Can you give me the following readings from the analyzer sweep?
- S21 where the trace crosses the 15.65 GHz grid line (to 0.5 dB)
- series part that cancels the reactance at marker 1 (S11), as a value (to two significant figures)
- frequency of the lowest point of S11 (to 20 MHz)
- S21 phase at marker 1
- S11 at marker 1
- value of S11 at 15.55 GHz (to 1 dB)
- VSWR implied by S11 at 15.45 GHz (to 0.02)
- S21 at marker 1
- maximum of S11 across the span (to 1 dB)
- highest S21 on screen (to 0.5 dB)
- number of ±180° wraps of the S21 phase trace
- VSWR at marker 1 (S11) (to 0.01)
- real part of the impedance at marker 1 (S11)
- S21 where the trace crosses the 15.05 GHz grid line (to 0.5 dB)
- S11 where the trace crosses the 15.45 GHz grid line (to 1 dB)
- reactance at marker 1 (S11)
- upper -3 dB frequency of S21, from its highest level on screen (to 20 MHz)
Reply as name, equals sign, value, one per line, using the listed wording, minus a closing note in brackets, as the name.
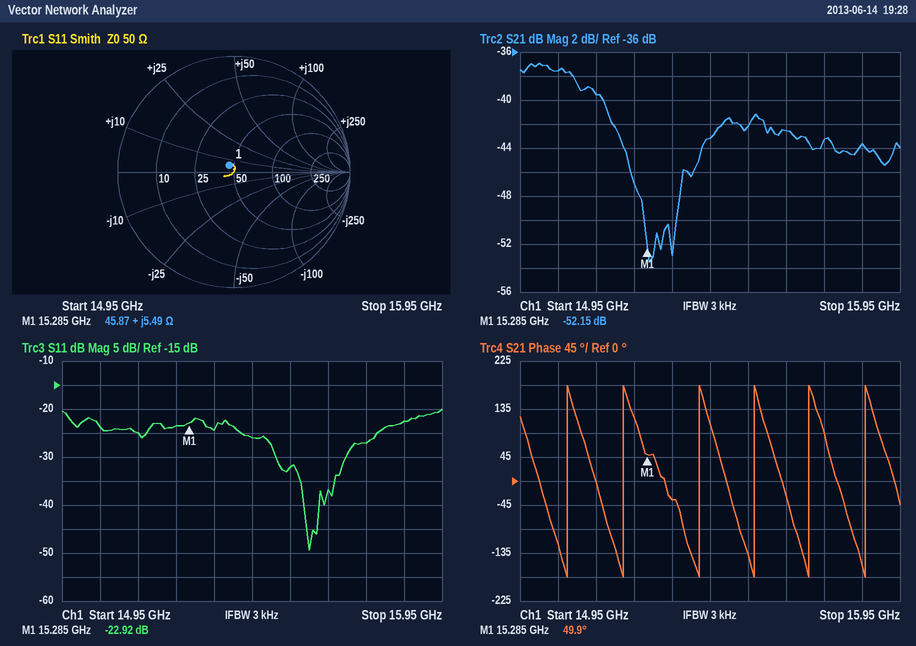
S21 where the trace crosses the 15.65 GHz grid line = -42.5 dB
series part that cancels the reactance at marker 1 (S11), as a value = 1.9 pF
frequency of the lowest point of S11 = 15.60 GHz
S21 phase at marker 1 = 49.9°
S11 at marker 1 = -22.92 dB
value of S11 at 15.55 GHz = -32 dB
VSWR implied by S11 at 15.45 GHz = 1.10
S21 at marker 1 = -52.15 dB
maximum of S11 across the span = -20 dB
highest S21 on screen = -37.0 dB
number of ±180° wraps of the S21 phase trace = 6
VSWR at marker 1 (S11) = 1.15
real part of the impedance at marker 1 = 45.87 Ω
S21 where the trace crosses the 15.05 GHz grid line = -37.5 dB
S11 where the trace crosses the 15.45 GHz grid line = -26 dB
reactance at marker 1 = +5.49 Ω
upper -3 dB frequency of S21, from its highest level on screen = 15.16 GHz
